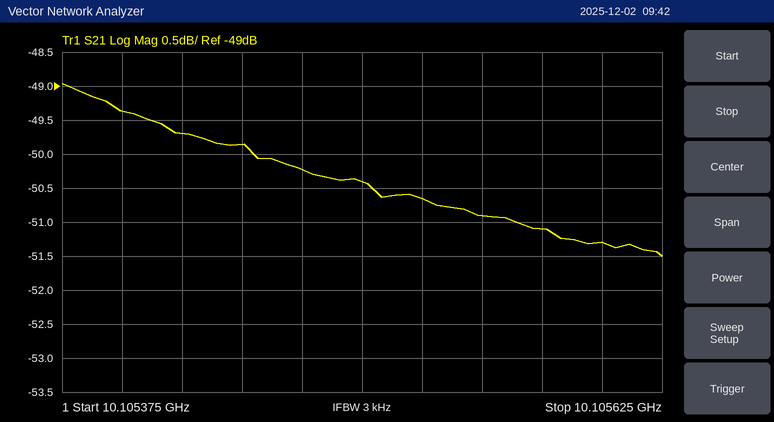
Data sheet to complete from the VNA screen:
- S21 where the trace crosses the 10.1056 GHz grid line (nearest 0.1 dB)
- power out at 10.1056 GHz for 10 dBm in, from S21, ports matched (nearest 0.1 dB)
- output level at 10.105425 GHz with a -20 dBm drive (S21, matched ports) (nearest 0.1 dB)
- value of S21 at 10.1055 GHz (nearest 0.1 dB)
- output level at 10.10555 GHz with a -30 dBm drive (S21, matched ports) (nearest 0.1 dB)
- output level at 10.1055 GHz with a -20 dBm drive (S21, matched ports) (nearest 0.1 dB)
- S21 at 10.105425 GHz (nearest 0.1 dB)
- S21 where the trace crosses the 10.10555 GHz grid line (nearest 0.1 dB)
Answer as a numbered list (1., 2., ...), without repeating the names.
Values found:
1. -51.3 dB
2. -41.3 dBm
3. -69.7 dBm
4. -50.4 dB
5. -80.9 dBm
6. -70.4 dBm
7. -49.7 dB
8. -50.9 dB
